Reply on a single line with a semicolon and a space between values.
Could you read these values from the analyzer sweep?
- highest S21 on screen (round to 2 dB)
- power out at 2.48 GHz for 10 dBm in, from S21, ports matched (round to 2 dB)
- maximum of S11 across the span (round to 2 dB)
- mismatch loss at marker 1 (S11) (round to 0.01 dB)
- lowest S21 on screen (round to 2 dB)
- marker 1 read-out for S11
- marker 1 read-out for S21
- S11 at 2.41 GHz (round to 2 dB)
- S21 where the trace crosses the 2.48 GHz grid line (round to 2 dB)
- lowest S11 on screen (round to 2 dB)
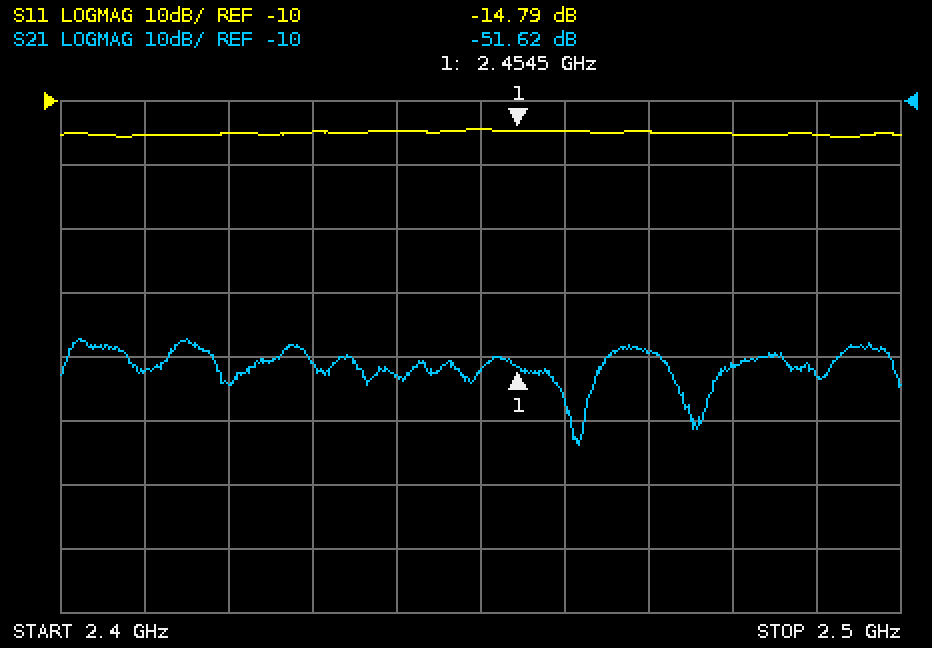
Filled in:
-48 dB; -42 dBm; -14 dB; 0.15 dB; -64 dB; -14.79 dB; -51.62 dB; -16 dB; -52 dB; -16 dB
